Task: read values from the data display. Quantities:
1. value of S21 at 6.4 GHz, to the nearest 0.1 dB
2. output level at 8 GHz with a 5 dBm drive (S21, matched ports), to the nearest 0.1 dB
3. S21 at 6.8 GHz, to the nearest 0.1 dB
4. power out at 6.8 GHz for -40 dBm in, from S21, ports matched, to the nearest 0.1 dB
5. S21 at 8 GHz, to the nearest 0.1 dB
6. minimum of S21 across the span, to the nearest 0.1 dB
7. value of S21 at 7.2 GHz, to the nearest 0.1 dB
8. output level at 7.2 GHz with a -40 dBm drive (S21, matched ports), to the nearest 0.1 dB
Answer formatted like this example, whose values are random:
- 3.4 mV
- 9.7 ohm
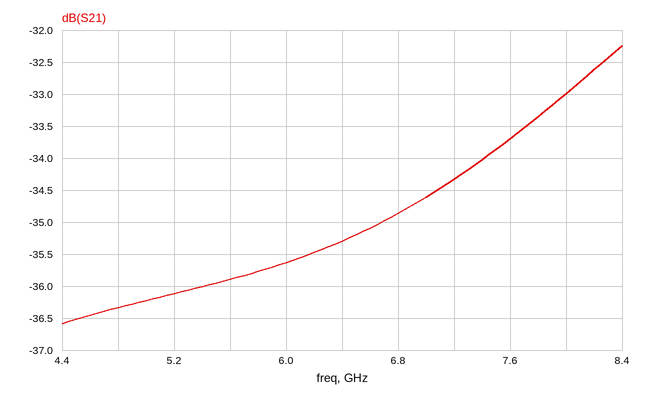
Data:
- -35.3 dB
- -28.0 dBm
- -34.9 dB
- -74.9 dBm
- -33.0 dB
- -36.6 dB
- -34.3 dB
- -74.3 dBm
